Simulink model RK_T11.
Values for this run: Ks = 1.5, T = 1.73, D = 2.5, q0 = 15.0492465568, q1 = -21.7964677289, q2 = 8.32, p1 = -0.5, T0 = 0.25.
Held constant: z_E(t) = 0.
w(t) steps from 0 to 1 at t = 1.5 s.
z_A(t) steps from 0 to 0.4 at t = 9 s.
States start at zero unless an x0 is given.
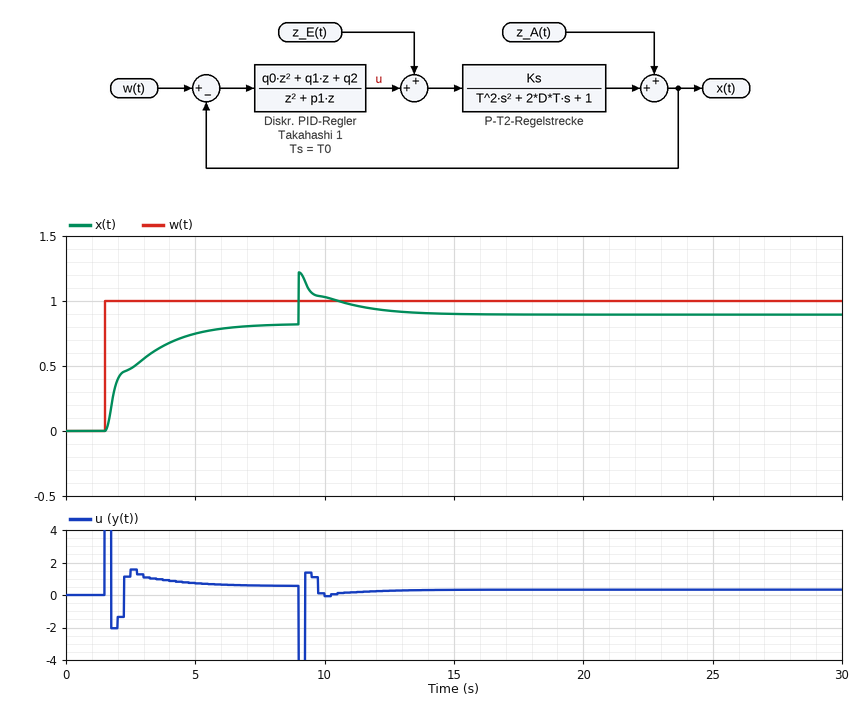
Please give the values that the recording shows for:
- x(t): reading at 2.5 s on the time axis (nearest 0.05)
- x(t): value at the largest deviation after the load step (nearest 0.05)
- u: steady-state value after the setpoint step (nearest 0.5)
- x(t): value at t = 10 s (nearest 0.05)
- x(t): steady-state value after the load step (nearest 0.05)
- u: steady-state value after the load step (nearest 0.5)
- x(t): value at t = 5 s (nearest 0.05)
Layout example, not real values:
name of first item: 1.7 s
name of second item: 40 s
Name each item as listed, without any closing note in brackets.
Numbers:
x(t): reading at 2.5 s on the time axis: 0.50
x(t): value at the largest deviation after the load step: 1.20
u: steady-state value after the setpoint step: 0.5
x(t): value at t = 10 s: 1.05
x(t): steady-state value after the load step: 0.90
u: steady-state value after the load step: 0.5
x(t): value at t = 5 s: 0.75
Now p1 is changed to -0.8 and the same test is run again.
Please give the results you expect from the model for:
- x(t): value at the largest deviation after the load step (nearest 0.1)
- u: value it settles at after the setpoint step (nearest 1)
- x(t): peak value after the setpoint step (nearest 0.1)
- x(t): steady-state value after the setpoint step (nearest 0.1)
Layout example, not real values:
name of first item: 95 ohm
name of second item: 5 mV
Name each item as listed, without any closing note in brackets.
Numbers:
x(t): value at the largest deviation after the load step: 1.3
u: value it settles at after the setpoint step: 1
x(t): peak value after the setpoint step: 1.0
x(t): steady-state value after the setpoint step: 0.9
